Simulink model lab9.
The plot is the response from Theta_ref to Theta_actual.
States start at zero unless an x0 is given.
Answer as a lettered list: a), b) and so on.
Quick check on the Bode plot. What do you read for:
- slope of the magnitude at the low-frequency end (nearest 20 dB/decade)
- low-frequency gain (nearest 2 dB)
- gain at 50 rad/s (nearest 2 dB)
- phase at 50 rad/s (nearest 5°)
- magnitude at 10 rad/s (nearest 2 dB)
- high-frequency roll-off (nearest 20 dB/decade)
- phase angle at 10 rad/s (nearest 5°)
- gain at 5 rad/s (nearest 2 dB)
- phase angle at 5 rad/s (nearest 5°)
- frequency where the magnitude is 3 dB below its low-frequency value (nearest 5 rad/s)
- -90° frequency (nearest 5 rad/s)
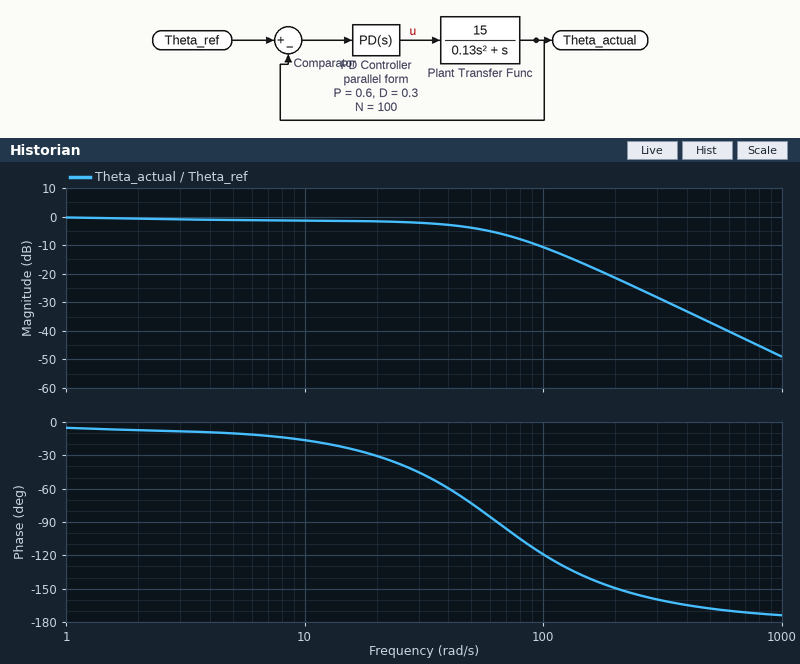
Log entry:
a) 0 dB/decade
b) 0 dB
c) -4 dB
d) -75°
e) -2 dB
f) -40 dB/decade
g) -15°
h) -2 dB
i) -10°
j) 45 rad/s
k) 65 rad/s
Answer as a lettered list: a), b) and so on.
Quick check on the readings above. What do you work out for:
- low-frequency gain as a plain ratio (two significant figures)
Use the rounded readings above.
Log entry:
a) 1.0
